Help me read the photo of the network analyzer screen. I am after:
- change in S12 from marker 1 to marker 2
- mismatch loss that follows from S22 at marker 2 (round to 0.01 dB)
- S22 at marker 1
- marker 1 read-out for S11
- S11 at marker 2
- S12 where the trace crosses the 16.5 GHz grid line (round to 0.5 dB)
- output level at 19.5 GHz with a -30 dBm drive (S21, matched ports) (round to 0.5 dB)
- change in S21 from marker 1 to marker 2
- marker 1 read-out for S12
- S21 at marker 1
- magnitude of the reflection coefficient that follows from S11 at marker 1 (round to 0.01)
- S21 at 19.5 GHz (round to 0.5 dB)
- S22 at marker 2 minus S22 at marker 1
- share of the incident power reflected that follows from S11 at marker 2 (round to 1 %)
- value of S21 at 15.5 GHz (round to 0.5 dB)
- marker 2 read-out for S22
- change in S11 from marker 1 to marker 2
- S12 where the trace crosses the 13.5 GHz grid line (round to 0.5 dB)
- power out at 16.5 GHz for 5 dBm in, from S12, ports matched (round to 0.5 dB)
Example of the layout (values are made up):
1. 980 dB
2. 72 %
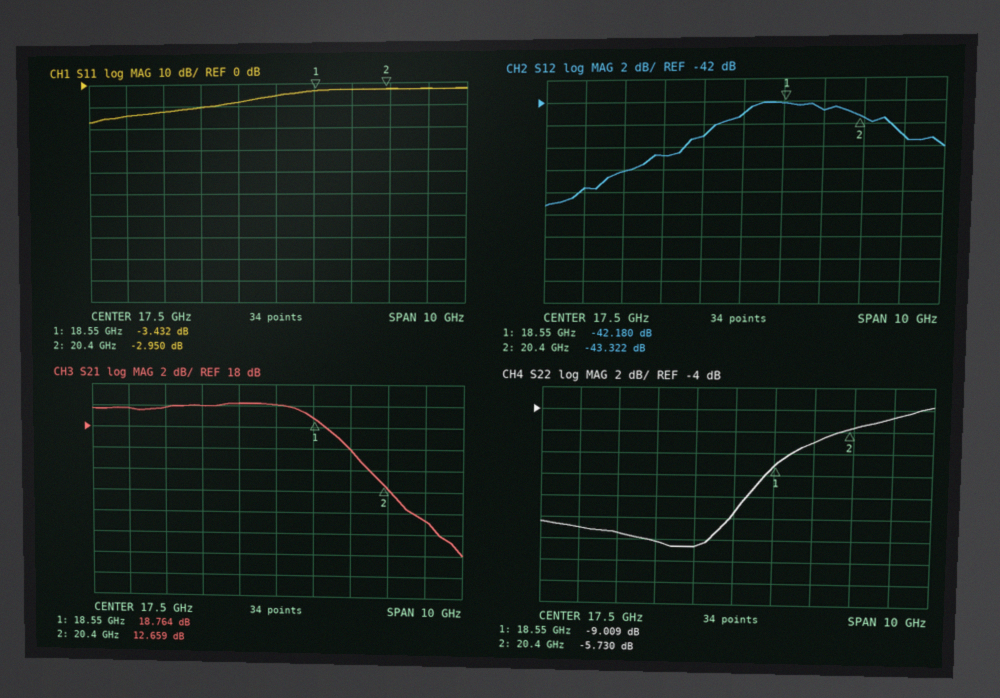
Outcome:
1. -1.142 dB
2. 1.35 dB
3. -9.009 dB
4. -3.432 dB
5. -2.950 dB
6. -45.0 dB
7. -14.0 dBm
8. -6.105 dB
9. -42.180 dB
10. 18.764 dB
11. 0.67
12. 16.0 dB
13. 3.279 dB
14. 51 %
15. 20.0 dB
16. -5.730 dB
17. 0.482 dB
18. -49.5 dB
19. -40.0 dBm
